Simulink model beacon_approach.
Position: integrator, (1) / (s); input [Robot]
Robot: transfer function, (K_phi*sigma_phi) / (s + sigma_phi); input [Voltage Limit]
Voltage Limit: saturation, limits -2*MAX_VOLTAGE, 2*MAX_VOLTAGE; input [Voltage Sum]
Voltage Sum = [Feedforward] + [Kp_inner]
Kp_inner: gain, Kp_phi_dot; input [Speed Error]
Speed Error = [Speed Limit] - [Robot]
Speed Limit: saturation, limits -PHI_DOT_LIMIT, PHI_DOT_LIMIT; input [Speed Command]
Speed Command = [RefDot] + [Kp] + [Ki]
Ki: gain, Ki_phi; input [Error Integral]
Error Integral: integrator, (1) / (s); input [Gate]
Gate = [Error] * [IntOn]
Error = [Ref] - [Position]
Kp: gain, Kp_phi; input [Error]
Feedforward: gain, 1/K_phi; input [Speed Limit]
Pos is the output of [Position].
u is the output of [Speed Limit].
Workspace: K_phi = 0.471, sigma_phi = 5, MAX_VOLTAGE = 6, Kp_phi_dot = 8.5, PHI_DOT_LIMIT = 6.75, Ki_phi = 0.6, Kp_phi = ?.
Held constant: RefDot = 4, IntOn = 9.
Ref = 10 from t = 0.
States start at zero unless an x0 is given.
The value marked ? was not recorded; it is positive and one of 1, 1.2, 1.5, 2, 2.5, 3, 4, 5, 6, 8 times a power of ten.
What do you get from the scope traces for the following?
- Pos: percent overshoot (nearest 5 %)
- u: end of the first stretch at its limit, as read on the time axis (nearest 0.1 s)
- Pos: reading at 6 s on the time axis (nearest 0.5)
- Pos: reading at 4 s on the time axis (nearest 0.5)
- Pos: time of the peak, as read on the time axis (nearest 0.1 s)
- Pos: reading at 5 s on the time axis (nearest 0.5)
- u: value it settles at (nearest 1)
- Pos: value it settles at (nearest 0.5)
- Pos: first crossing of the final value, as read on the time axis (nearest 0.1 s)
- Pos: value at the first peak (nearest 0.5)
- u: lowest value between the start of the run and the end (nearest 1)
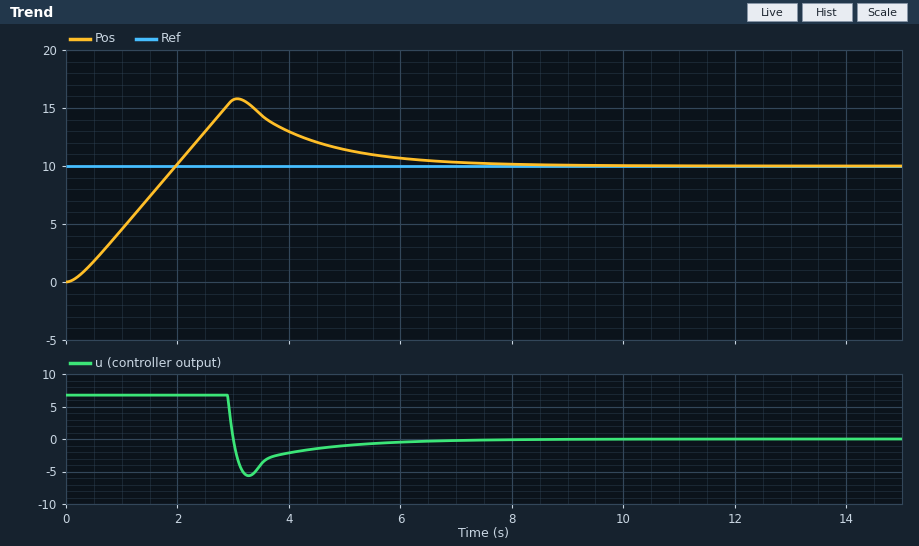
60 %
2.9 s
10.5
13.0
3.1 s
11.5
0
10.0
2.0 s
16.0
-6
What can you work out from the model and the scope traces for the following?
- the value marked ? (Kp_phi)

8
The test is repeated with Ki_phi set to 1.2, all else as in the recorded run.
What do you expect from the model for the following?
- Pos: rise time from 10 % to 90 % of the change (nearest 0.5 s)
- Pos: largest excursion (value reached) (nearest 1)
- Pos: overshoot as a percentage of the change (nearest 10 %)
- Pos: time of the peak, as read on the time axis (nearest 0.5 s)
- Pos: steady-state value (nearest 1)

1.5 s
18
80 %
3.5 s
10
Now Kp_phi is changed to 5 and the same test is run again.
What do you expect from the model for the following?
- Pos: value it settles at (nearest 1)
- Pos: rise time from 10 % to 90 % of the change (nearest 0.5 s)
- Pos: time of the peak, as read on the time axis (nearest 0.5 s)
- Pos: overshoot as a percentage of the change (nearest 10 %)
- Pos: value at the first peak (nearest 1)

10
1.5 s
3.5 s
70 %
17
